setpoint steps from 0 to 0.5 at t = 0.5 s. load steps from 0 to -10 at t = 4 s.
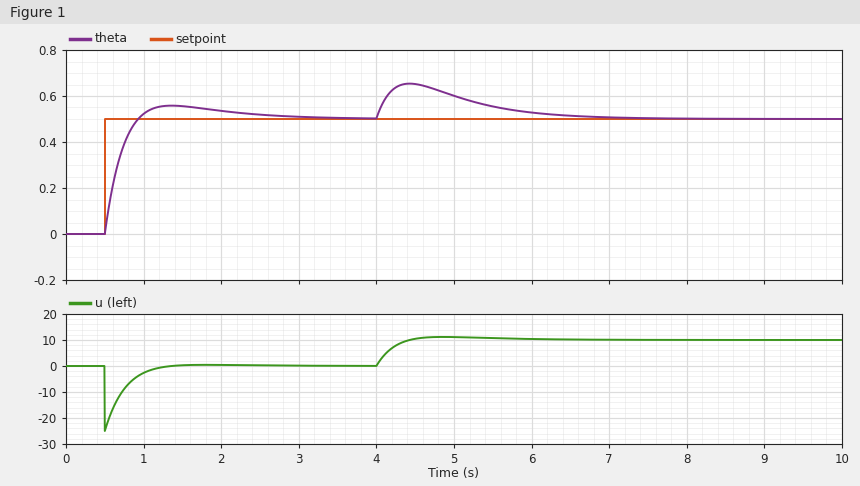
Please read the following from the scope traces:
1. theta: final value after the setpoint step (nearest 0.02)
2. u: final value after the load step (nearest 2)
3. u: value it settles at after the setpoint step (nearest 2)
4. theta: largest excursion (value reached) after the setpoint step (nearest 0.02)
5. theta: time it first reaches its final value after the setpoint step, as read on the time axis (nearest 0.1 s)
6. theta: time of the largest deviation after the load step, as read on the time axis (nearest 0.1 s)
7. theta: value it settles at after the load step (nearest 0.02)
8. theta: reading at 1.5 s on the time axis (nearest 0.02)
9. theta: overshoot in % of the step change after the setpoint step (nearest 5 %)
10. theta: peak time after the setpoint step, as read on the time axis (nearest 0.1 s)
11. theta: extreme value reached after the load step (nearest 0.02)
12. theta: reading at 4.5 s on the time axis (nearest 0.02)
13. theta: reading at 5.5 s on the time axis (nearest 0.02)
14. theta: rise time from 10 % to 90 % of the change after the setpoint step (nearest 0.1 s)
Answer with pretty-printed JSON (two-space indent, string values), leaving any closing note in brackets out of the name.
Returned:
{
  "theta: final value after the setpoint step": "0.50",
  "u: final value after the load step": "10",
  "u: value it settles at after the setpoint step": "0",
  "theta: largest excursion (value reached) after the setpoint step": "0.56",
  "theta: time it first reaches its final value after the setpoint step, as read on the time axis": "0.9 s",
  "theta: time of the largest deviation after the load step, as read on the time axis": "4.4 s",
  "theta: value it settles at after the load step": "0.50",
  "theta: reading at 1.5 s on the time axis": "0.56",
  "theta: overshoot in % of the step change after the setpoint step": "10 %",
  "theta: peak time after the setpoint step, as read on the time axis": "1.4 s",
  "theta: extreme value reached after the load step": "0.66",
  "theta: reading at 4.5 s on the time axis": "0.66",
  "theta: reading at 5.5 s on the time axis": "0.56",
  "theta: rise time from 10 % to 90 % of the change after the setpoint step": "0.3 s"
}
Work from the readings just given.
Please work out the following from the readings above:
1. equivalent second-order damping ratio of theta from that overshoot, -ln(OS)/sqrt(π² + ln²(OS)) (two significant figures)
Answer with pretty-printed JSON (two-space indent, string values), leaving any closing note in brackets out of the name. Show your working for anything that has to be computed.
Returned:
{
  "equivalent second-order damping ratio of theta from that overshoot, -ln(OS)/sqrt(π² + ln²(OS))": "ln(0.1) = -2.303; 2.303 / sqrt(9.870 + 5.302) = 0.59"
}
